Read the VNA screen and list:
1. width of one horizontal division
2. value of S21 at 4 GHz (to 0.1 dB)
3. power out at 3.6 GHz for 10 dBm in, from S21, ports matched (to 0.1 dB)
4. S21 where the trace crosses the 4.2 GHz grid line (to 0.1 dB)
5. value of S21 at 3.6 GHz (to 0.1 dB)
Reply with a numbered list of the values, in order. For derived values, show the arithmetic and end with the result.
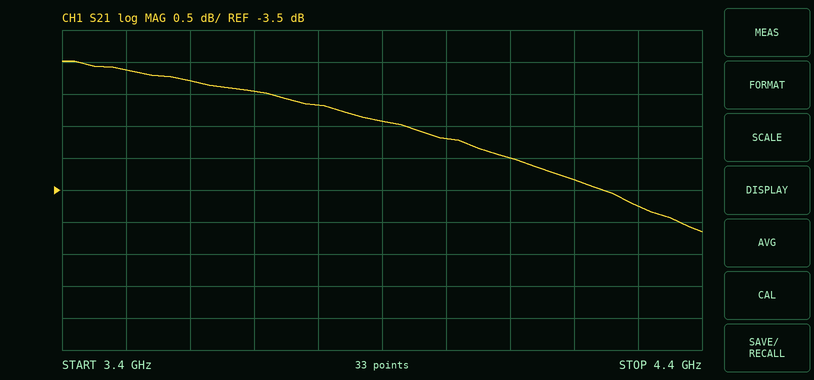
1. 100 MHz
2. -2.7 dB
3. 10 dBm + (-1.8 dB) = 8.2 dBm
4. -3.3 dB
5. -1.8 dB
